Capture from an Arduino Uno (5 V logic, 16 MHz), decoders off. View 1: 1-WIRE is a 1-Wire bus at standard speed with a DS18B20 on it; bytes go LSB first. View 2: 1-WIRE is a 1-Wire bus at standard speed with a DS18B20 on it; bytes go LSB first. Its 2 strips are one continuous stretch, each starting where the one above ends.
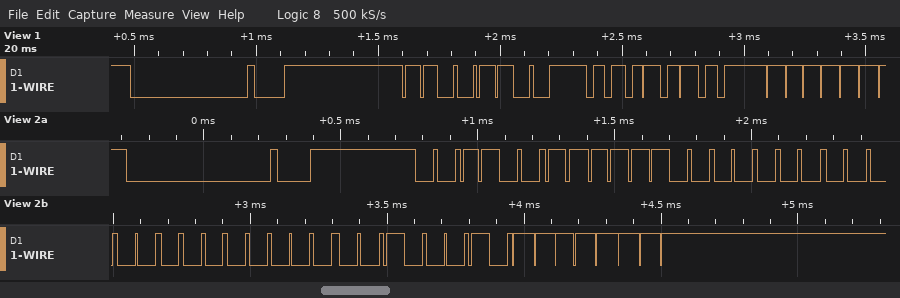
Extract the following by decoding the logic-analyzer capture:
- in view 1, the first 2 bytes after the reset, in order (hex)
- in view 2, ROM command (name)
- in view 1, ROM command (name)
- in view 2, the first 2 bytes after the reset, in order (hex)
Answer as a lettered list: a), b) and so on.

a) 33 28
b) Skip ROM
c) Read ROM
d) CC 0F
